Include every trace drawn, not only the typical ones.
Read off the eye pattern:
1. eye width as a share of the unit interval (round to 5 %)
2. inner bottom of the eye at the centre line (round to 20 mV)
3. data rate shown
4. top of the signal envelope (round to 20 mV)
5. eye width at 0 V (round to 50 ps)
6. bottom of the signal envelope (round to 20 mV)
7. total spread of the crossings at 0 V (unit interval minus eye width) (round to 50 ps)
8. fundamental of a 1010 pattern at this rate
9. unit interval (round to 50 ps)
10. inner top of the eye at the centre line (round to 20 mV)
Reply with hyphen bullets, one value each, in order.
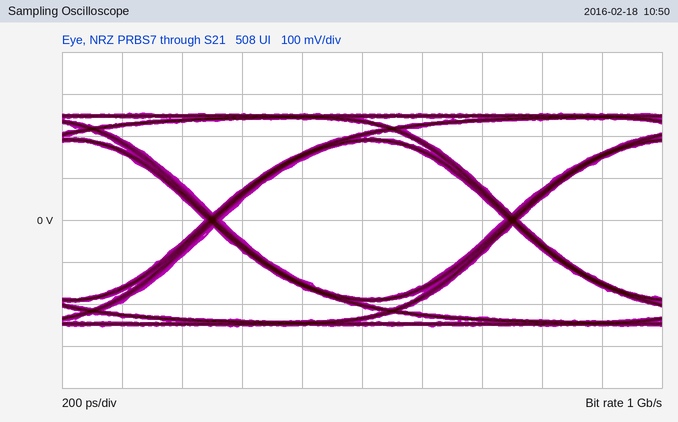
- 95 %
- -180 mV
- 1 Gb/s
- 260 mV
- 950 ps
- -260 mV
- 50 ps
- 500 MHz
- 1.00 ns
- 180 mV
